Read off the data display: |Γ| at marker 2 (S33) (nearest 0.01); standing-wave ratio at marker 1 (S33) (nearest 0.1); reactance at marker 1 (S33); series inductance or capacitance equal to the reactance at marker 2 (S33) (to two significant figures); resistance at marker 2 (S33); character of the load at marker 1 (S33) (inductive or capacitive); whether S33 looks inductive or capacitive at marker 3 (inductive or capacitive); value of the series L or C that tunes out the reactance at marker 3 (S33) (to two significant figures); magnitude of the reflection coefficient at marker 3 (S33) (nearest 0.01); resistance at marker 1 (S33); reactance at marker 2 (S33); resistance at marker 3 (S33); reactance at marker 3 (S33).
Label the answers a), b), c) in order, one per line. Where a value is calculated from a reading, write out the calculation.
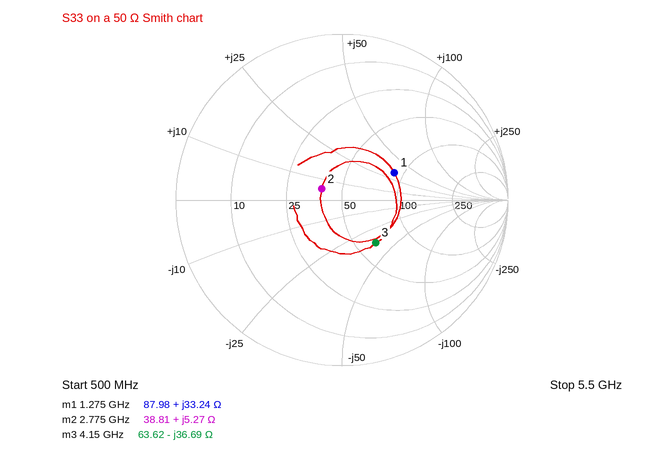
a) 0.14
b) 2.1
c) +33.24 Ω
d) L = 5.27 Ω/(2π × 2.775 GHz) ≈ 302 pH, so 300 pH to two significant figures
e) 38.81 Ω
f) inductive
g) capacitive
h) L = 36.69 Ω/(2π × 4.15 GHz) ≈ 1.4 nH
i) 0.33
j) 87.98 Ω
k) +5.27 Ω
l) 63.62 Ω
m) -36.69 Ω
